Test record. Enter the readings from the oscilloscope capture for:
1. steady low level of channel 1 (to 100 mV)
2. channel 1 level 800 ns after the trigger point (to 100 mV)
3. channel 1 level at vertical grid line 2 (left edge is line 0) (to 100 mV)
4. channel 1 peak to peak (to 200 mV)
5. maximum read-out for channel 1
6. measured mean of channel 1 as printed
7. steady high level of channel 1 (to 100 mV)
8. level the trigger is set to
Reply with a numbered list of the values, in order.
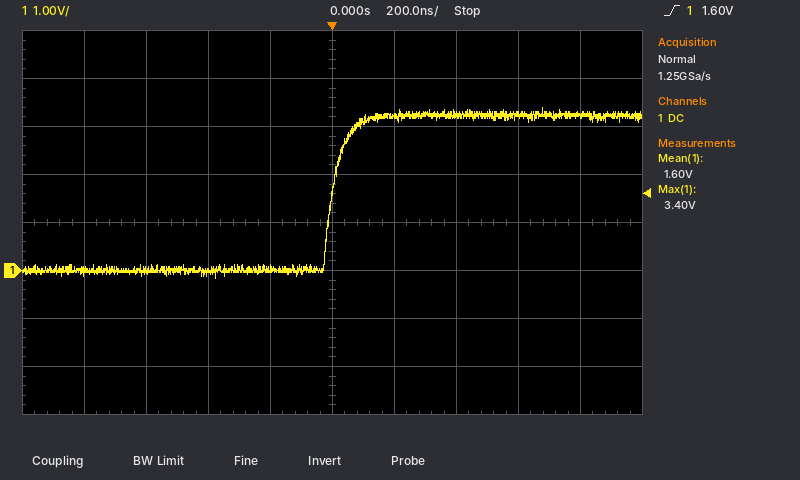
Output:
1. 0.0 V
2. 3.2 V
3. 0.0 V
4. 3.6 V
5. 3.40 V
6. 1.60 V
7. 3.2 V
8. 1.60 V
